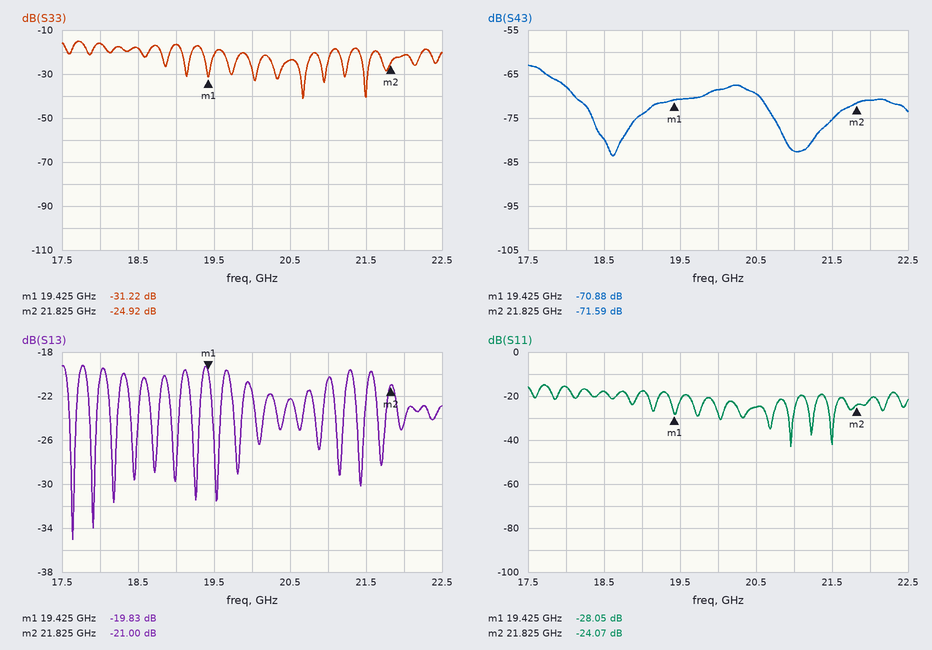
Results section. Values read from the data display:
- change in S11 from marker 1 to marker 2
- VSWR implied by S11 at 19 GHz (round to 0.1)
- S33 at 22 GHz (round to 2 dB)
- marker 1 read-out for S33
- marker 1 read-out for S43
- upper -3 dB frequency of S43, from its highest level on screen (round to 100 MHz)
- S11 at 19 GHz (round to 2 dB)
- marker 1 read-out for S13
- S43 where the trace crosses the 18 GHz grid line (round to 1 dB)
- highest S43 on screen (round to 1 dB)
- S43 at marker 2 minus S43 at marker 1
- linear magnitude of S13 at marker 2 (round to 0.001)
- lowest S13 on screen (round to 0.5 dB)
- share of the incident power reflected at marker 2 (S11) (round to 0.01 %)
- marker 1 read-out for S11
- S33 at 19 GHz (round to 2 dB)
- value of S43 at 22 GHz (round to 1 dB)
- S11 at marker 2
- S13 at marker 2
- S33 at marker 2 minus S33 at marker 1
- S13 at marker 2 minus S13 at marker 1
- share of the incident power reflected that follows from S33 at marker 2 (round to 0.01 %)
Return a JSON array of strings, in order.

["3.98 dB", "1.3", "-22 dB", "-31.22 dB", "-70.88 dB", "17.8 GHz", "-18 dB", "-19.83 dB", "-68 dB", "-63 dB", "-0.71 dB", "0.089", "-35.0 dB", "0.39 %", "-28.05 dB", "-16 dB", "-71 dB", "-24.07 dB", "-21.00 dB", "6.30 dB", "-1.17 dB", "0.32 %"]
